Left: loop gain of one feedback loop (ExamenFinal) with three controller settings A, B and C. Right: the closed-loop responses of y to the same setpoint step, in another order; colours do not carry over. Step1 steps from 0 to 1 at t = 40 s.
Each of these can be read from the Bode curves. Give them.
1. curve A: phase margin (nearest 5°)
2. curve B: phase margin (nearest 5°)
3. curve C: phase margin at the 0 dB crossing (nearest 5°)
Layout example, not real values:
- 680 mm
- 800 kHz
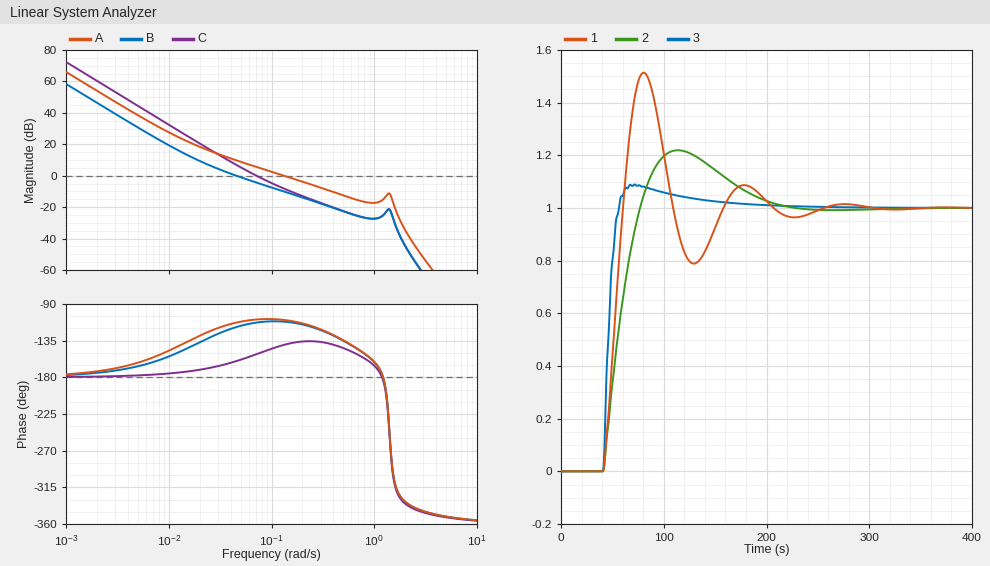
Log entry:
- 70°
- 60°
- 30°
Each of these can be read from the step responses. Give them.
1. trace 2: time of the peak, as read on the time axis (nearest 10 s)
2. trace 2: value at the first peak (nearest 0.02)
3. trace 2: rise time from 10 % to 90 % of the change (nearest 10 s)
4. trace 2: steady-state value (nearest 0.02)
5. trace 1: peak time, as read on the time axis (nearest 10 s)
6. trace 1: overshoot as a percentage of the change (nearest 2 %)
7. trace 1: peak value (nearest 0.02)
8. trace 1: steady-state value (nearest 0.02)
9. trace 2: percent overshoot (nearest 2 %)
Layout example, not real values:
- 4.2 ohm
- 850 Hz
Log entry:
- 110 s
- 1.22
- 30 s
- 1.00
- 80 s
- 52 %
- 1.52
- 1.00
- 22 %
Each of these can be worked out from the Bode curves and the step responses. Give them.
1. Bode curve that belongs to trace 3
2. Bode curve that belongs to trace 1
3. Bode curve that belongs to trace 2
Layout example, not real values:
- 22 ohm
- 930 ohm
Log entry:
- A
- C
- B
